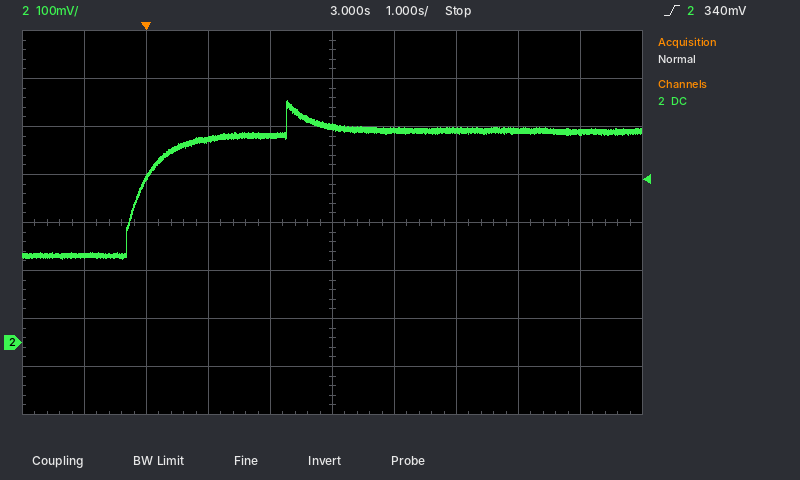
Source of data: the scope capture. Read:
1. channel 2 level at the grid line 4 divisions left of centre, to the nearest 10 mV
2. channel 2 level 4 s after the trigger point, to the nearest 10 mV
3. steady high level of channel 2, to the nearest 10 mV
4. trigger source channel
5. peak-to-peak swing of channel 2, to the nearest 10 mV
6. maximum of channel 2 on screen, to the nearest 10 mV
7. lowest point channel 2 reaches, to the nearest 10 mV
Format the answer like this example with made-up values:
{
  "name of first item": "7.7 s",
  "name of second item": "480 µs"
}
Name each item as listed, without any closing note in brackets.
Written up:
{
  "channel 2 level at the grid line 4 divisions left of centre, to the nearest 10 mV": "180 mV",
  "channel 2 level 4 s after the trigger point, to the nearest 10 mV": "440 mV",
  "steady high level of channel 2, to the nearest 10 mV": "440 mV",
  "trigger source channel": "channel 2",
  "peak-to-peak swing of channel 2, to the nearest 10 mV": "330 mV",
  "maximum of channel 2 on screen, to the nearest 10 mV": "500 mV",
  "lowest point channel 2 reaches, to the nearest 10 mV": "170 mV"
}
